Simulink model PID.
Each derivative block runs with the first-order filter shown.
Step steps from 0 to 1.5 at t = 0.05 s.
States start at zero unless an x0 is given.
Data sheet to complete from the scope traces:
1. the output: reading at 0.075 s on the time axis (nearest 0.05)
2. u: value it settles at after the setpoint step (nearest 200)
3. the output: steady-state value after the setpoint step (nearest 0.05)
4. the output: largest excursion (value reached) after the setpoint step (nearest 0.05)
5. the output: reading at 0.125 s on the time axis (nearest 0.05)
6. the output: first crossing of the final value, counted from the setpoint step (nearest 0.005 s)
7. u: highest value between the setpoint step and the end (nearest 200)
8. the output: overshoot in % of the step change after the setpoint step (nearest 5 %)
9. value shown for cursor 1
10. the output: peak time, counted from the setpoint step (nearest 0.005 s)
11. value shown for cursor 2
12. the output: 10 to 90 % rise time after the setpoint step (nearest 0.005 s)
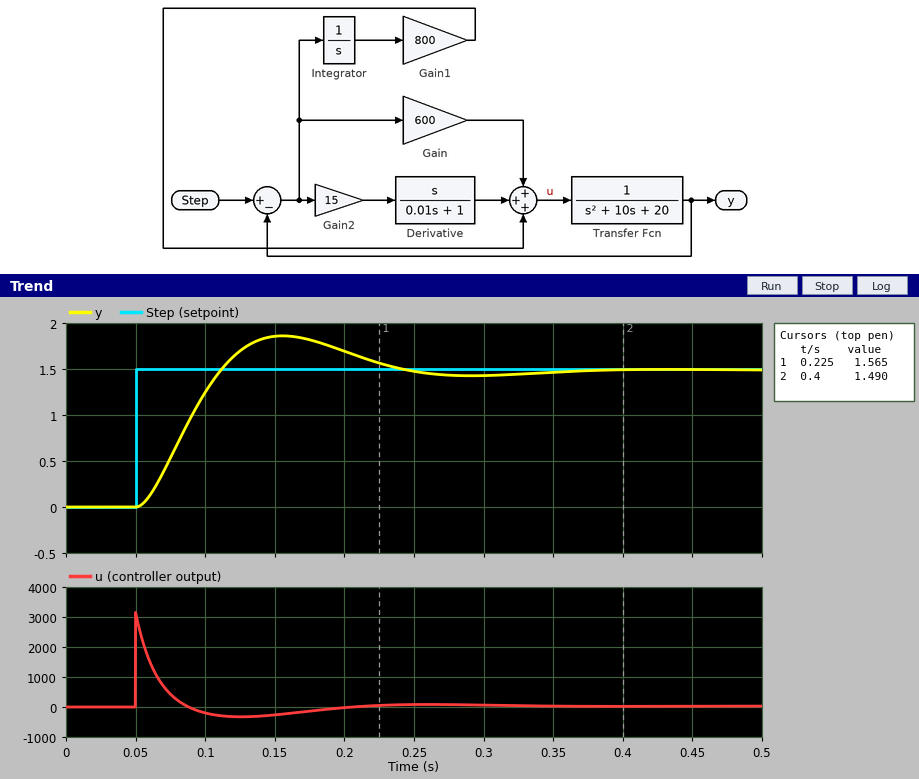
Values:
0.55
0
1.50
1.85
1.70
0.060 s
3200
25 %
1.565
0.105 s
1.490
0.045 s
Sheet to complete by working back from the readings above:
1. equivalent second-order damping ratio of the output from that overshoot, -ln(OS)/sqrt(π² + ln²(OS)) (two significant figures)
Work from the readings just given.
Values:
0.40
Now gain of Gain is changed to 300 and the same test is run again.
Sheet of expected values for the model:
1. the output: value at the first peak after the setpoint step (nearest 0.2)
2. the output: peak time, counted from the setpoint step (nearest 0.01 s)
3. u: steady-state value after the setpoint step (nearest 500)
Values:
1.6
0.16 s
0
